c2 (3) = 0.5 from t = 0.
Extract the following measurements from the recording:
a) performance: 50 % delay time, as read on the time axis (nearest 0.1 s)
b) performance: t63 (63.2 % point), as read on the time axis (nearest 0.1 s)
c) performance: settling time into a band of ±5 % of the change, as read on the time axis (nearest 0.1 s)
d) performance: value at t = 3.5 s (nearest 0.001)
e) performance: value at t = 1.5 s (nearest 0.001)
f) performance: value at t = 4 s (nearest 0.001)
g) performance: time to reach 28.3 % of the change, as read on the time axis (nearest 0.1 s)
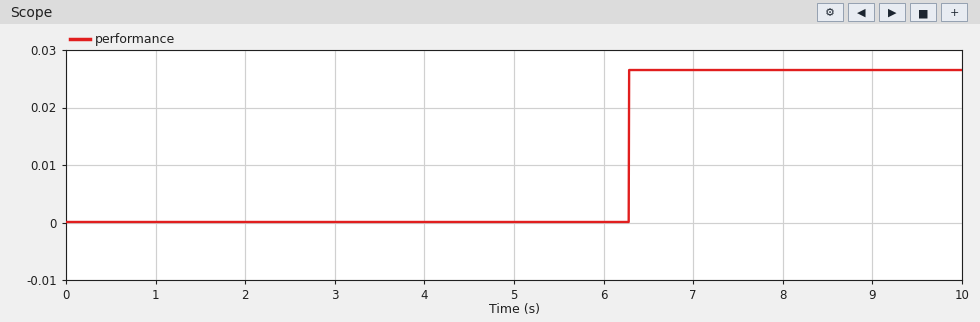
6.3 s
6.3 s
6.3 s
0.000
0.000
0.000
6.3 s
